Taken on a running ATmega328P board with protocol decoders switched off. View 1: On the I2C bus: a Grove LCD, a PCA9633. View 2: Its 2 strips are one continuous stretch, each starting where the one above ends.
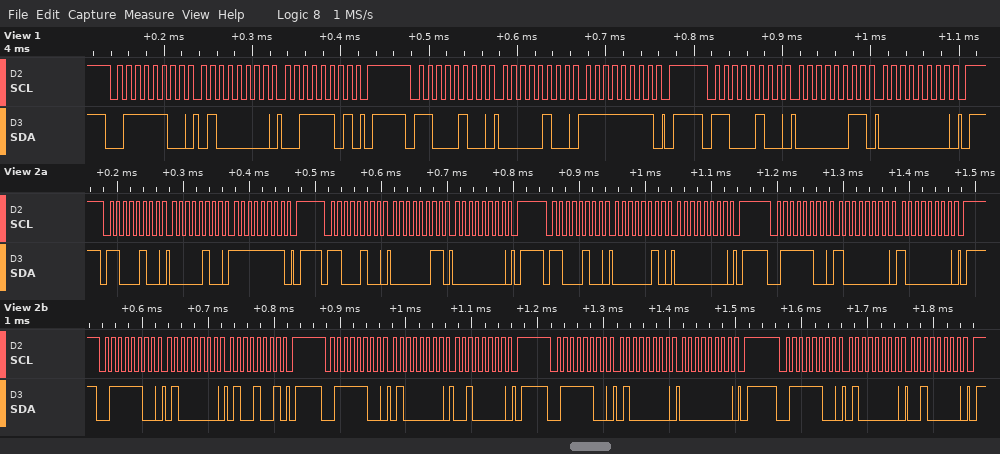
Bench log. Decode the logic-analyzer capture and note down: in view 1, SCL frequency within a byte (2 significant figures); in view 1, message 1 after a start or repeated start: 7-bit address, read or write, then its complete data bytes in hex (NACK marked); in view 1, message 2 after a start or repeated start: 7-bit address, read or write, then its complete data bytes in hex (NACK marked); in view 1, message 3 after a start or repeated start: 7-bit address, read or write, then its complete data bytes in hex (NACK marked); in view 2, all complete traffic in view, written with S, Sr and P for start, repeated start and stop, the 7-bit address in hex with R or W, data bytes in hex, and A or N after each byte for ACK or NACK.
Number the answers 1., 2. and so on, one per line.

1. 100 kHz
2. 0x3E write: 40 3D
3. 0x62 write: 04 FF
4. 0x62 write: 03 00
5. S 62W A 04 A FF A P S 62W A 03 A 00 A P S 62W A 02 A 00 A P S 3EW A 80 A 80 A P S 3EW A 40 A 49 A P S 3EW A 40 A 20 A P S 3EW A 40 A 00 A P S 3EW A 40 A 20 A P
